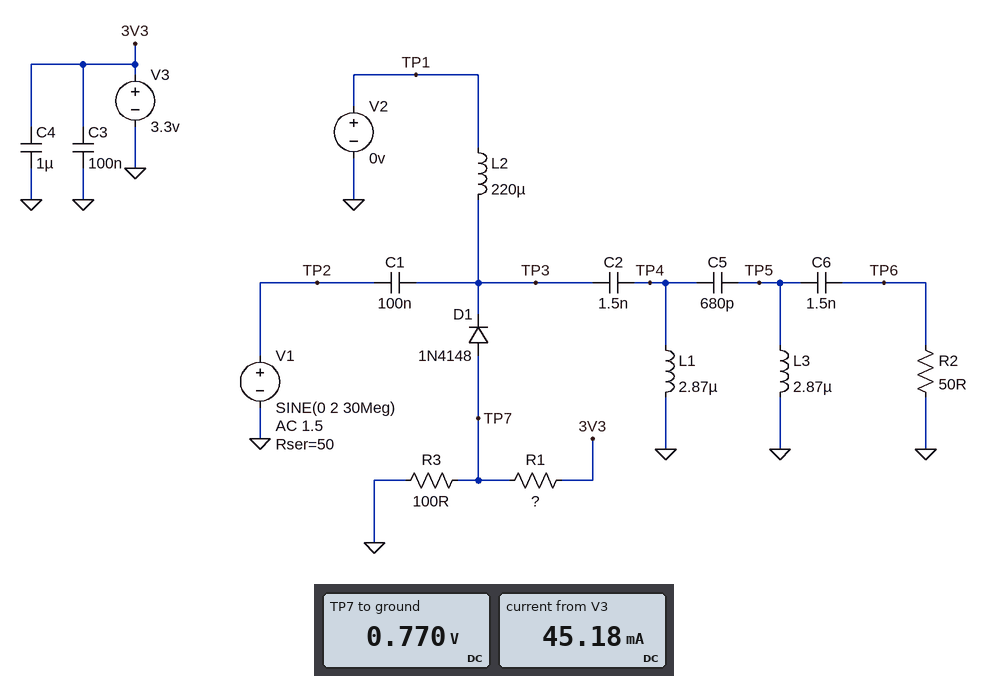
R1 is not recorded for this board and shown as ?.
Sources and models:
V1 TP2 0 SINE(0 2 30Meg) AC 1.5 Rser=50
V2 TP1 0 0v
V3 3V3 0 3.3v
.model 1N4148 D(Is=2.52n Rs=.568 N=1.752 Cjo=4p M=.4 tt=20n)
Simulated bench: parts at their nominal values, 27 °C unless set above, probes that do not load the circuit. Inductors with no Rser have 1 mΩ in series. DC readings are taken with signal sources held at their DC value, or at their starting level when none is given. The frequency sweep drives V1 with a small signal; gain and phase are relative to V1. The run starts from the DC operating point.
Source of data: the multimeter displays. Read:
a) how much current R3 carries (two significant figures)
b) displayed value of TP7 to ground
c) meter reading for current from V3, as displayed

7.7 mA
0.770 V
45.18 mA
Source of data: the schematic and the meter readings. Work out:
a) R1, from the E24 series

56 Ω
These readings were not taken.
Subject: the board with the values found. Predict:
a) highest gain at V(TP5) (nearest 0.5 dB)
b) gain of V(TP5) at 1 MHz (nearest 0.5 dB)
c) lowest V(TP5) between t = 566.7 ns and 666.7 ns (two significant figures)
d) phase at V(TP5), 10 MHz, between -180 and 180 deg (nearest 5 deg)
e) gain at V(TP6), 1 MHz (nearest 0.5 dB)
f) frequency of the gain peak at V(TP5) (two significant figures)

-6.5 dB
-40.5 dB
-590 mV
30 deg
-48.0 dB
2.0 MHz
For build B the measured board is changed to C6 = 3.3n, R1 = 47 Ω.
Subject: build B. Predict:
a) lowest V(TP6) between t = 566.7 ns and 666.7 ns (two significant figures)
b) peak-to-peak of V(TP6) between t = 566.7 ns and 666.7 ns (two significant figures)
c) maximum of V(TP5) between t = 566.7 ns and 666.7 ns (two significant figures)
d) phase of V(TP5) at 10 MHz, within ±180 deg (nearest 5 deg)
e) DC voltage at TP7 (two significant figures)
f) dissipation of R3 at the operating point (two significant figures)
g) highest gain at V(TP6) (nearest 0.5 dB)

-560 mV
1.1 V
570 mV
35 deg
780 mV
6.1 mW
-10.5 dB
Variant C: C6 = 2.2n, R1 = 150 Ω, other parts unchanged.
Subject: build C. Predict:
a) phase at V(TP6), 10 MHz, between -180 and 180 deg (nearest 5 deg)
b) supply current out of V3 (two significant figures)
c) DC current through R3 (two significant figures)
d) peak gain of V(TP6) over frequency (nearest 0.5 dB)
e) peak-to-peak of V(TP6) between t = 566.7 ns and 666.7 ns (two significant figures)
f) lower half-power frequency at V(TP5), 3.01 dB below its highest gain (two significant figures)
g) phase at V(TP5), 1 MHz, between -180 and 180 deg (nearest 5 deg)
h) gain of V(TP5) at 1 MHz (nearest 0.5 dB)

40 deg
17 mA
7.0 mA
-9.0 dB
1.4 V
1.8 MHz
-25 deg
-38.0 dB
